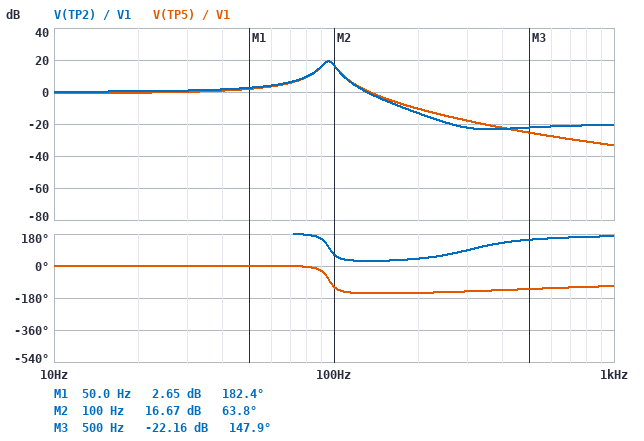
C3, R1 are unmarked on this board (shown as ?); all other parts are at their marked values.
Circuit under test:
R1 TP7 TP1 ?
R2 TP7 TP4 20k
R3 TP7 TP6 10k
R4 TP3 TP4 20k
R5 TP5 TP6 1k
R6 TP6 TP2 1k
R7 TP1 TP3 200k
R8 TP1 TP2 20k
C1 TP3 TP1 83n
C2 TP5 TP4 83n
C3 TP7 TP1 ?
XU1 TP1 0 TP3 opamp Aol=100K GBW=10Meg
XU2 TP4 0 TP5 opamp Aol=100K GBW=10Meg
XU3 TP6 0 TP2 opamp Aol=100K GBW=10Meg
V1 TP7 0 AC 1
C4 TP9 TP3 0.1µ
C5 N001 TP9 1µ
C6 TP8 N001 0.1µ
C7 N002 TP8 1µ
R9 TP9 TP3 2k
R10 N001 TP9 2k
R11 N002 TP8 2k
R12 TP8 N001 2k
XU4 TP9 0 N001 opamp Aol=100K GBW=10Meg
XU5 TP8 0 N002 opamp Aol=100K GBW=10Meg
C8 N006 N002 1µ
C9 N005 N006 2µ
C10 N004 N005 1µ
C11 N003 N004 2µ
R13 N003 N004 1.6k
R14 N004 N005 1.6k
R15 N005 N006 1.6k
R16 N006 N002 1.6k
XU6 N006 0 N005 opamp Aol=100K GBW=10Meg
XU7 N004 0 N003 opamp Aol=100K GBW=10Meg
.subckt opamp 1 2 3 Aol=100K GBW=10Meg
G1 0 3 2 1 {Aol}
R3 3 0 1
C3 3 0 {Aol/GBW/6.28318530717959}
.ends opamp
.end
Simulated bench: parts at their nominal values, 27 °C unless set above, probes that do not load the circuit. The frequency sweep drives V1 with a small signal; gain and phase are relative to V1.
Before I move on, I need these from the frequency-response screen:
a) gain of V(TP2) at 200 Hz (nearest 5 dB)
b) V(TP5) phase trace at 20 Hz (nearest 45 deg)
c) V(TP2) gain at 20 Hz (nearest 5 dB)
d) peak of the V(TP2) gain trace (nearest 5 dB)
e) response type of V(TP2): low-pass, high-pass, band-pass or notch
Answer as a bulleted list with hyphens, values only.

- -15 dB
- 0 deg
- 0 dB
- 20 dB
- band-pass
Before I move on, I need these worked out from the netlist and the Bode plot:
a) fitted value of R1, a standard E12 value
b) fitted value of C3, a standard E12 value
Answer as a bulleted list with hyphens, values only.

- 18 kΩ
- 100 nF
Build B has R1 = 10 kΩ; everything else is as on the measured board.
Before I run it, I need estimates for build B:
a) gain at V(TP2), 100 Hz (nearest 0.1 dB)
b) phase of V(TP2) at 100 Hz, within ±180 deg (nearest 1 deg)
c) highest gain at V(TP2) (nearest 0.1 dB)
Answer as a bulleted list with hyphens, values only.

- 22.4 dB
- 57 deg
- 25.2 dB
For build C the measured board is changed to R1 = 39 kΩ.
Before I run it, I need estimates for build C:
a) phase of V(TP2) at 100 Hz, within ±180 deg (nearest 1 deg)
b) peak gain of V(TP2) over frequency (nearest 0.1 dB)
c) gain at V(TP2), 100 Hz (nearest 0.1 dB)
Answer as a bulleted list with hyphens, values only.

- 86 deg
- 11.6 dB
- 8.8 dB
